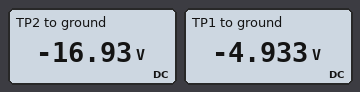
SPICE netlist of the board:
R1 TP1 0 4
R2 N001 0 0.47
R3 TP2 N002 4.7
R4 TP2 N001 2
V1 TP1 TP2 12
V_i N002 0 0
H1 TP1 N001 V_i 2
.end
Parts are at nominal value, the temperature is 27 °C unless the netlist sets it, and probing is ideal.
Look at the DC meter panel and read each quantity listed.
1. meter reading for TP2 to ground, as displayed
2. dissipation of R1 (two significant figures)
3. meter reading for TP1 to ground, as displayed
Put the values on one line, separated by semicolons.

-16.93 V; 6.1 W; -4.933 V
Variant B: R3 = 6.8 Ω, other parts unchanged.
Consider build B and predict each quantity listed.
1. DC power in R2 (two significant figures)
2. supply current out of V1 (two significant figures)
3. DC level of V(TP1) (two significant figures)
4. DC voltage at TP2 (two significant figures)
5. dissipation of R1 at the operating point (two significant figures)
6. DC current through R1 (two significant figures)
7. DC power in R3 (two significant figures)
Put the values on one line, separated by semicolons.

4.1 W; 10 A; -3.0 V; -15 V; 2.3 W; 760 mA; 33 W
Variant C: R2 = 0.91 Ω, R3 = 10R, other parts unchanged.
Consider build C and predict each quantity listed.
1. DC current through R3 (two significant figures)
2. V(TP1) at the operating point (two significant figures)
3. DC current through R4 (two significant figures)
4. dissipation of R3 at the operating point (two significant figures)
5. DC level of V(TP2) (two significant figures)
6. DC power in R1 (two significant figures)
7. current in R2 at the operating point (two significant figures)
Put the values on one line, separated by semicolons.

1.3 A; -1.2 V; 7.3 A; 17 W; -13 V; 340 mW; 1.6 A
